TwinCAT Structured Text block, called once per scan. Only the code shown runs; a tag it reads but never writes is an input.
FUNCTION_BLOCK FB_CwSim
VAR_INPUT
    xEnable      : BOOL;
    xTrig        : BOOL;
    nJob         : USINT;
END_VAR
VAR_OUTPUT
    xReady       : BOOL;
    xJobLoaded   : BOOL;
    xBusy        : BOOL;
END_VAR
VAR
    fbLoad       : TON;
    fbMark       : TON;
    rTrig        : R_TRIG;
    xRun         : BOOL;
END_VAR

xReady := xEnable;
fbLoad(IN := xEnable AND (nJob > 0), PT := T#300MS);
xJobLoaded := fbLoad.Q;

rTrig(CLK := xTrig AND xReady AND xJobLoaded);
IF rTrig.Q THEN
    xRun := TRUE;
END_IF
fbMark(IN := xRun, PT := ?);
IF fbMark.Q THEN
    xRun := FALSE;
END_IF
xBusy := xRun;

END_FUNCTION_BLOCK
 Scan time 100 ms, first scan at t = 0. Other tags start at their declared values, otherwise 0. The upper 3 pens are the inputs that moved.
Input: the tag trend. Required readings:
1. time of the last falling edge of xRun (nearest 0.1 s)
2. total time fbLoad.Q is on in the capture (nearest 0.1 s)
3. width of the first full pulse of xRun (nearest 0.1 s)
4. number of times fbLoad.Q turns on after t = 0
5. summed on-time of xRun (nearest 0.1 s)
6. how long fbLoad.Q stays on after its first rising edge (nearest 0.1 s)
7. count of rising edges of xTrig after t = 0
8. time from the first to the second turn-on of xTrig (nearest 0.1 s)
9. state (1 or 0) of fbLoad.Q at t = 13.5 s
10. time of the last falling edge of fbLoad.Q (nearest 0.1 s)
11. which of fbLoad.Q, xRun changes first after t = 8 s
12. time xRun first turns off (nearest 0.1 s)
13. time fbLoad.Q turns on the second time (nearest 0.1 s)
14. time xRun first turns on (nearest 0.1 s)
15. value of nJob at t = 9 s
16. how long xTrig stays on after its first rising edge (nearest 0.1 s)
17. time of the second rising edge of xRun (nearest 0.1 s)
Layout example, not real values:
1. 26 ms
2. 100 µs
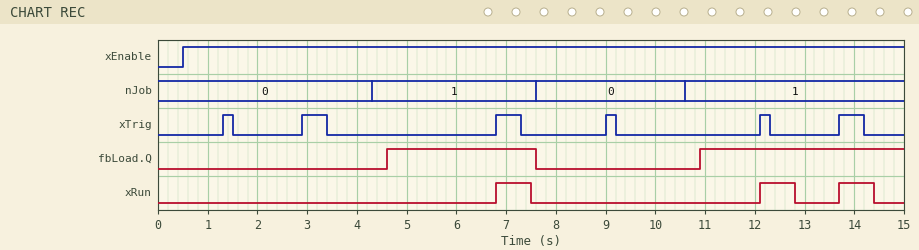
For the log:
1. 14.4 s
2. 7.1 s
3. 0.7 s
4. 2
5. 2.1 s
6. 3.0 s
7. 6
8. 1.6 s
9. 1
10. 7.6 s
11. fbLoad.Q
12. 7.5 s
13. 10.9 s
14. 6.8 s
15. 0
16. 0.2 s
17. 12.1 s
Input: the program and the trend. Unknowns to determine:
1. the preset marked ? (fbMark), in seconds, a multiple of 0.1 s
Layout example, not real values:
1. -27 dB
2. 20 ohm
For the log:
1. 0.7 s
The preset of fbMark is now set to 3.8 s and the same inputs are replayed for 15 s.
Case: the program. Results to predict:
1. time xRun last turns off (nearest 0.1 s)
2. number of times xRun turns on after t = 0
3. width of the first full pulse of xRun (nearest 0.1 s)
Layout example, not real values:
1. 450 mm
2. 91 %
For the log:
1. 10.6 s
2. 2
3. 3.8 s
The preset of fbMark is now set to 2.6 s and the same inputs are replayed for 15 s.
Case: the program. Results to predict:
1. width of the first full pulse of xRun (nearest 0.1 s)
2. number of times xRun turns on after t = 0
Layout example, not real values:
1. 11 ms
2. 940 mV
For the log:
1. 2.6 s
2. 2
